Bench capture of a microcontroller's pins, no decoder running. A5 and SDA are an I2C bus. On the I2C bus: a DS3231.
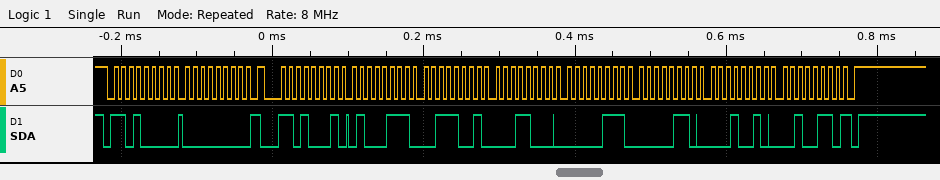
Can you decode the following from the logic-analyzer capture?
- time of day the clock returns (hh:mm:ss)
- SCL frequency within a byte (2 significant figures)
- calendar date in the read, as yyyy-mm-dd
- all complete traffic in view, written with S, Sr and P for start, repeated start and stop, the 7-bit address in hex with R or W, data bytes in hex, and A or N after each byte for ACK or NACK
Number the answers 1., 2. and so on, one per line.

1. 18:39:47
2. 100 kHz
3. 2026-12-06
4. S 68W A 00 A Sr 68R A 47 A 39 A 18 A 07 A 06 A 12 A 26 N P
